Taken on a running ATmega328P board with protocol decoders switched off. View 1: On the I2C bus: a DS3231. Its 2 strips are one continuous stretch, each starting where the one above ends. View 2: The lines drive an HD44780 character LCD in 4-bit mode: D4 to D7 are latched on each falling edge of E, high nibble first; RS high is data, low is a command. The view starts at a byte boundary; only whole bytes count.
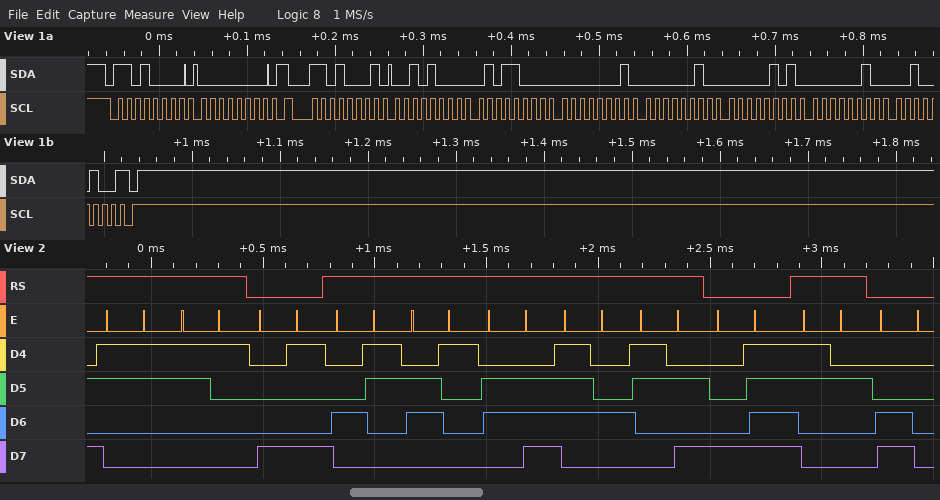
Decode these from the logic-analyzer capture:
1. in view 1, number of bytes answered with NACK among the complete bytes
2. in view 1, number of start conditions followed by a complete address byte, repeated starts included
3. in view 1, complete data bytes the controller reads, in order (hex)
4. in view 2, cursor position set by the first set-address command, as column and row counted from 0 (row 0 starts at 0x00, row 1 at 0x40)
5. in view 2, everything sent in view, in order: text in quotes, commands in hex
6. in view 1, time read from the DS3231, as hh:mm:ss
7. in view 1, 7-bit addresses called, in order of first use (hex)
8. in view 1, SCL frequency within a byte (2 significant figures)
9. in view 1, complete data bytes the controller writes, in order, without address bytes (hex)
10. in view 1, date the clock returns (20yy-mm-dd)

1
2
28 58 01 02 05 02 24
column 9, row 0
"31" 0x89 "Cant:" 0x8F "2" 0xC0
01:58:28
0x68
100 kHz
00
2024-02-05
